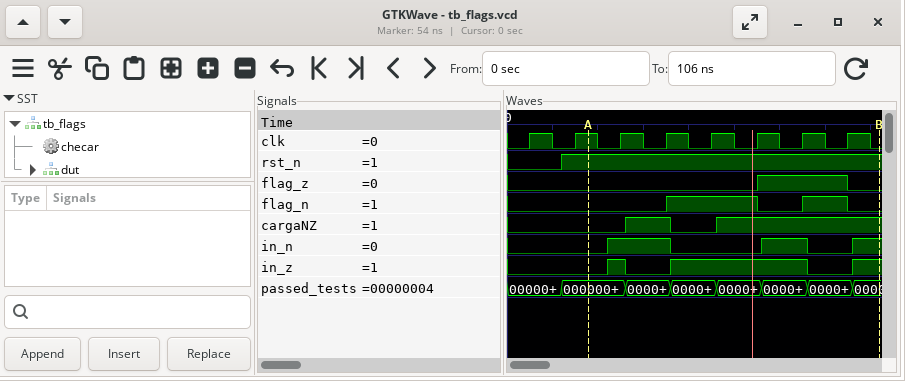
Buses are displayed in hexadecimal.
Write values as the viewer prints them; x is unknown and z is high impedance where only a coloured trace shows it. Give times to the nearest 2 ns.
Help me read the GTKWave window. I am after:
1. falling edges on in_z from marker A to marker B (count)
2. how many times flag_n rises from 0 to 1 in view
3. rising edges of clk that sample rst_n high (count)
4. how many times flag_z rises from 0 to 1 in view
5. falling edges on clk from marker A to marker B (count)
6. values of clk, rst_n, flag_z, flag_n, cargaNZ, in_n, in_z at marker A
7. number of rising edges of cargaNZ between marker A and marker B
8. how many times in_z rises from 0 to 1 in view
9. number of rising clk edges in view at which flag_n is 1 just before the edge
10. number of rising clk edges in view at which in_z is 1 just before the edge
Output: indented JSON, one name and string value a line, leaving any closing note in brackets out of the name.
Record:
{
  "falling edges on in_z from marker A to marker B": "2",
  "how many times flag_n rises from 0 to 1 in view": "2",
  "rising edges of clk that sample rst_n high": "7",
  "how many times flag_z rises from 0 to 1 in view": "1",
  "falling edges on clk from marker A to marker B": "7",
  "values of clk, rst_n, flag_z, flag_n, cargaNZ, in_n, in_z at marker A": "clk=1, rst_n=1, flag_z=0, flag_n=0, cargaNZ=0, in_n=0, in_z=0",
  "number of rising edges of cargaNZ between marker A and marker B": "2",
  "how many times in_z rises from 0 to 1 in view": "3",
  "number of rising clk edges in view at which flag_n is 1 just before the edge": "3",
  "number of rising clk edges in view at which in_z is 1 just before the edge": "4"
}
